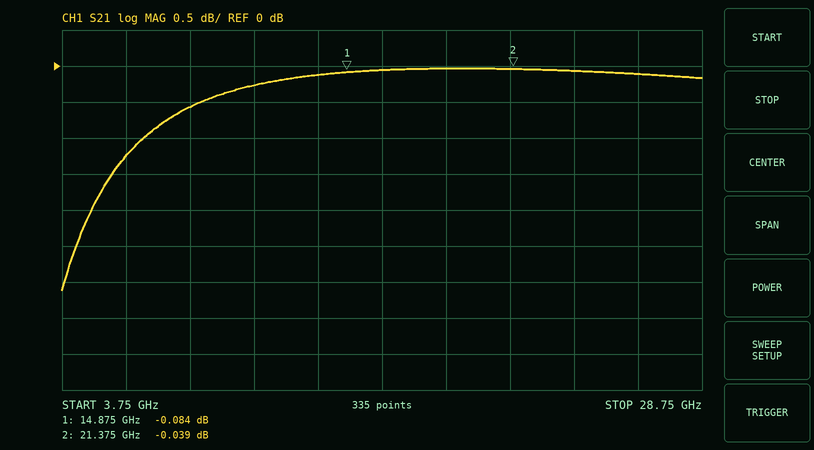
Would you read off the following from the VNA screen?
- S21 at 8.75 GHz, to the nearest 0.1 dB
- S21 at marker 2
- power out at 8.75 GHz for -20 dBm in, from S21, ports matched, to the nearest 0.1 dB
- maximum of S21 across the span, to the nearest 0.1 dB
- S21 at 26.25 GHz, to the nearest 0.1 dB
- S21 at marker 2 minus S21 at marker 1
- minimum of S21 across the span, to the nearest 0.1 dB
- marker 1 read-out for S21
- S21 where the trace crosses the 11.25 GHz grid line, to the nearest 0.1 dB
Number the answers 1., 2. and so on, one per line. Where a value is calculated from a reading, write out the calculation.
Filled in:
1. -0.6 dB
2. -0.039 dB
3. -20 dBm + (-0.6 dB) = -20.6 dBm
4. 0.0 dB
5. -0.1 dB
6. -0.039 − (-0.084) = 0.045 dB
7. -3.1 dB
8. -0.084 dB
9. -0.3 dB
